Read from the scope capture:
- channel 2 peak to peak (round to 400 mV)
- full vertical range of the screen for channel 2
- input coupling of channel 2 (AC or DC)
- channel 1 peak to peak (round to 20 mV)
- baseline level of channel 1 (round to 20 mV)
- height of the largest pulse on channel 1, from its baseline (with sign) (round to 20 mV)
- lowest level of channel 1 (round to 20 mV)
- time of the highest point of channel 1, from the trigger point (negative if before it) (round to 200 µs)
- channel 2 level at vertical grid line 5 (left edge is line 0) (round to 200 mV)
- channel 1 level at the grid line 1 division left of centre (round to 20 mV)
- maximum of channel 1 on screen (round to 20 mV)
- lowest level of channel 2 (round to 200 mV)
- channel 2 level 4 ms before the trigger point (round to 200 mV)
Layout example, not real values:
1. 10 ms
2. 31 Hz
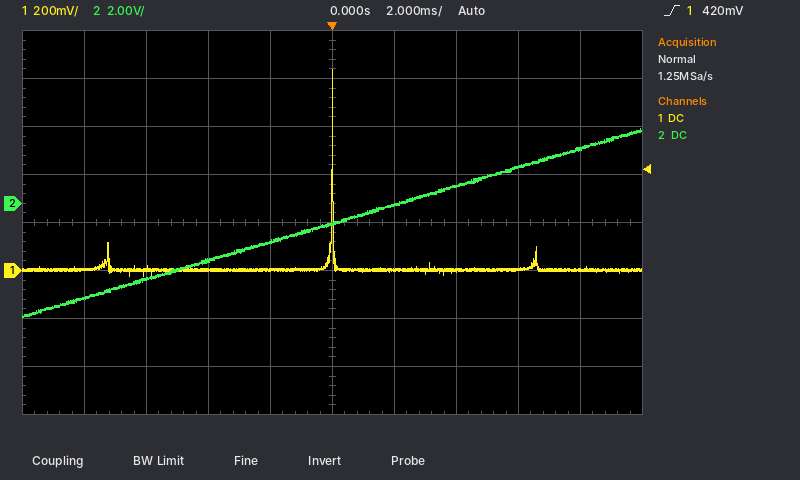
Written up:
1. 8.0 V
2. 16 V
3. DC
4. 860 mV
5. 0 mV
6. +840 mV
7. -20 mV
8. 0.0 ms
9. -800 mV
10. 0 mV
11. 840 mV
12. -4.8 V
13. -2.4 V
